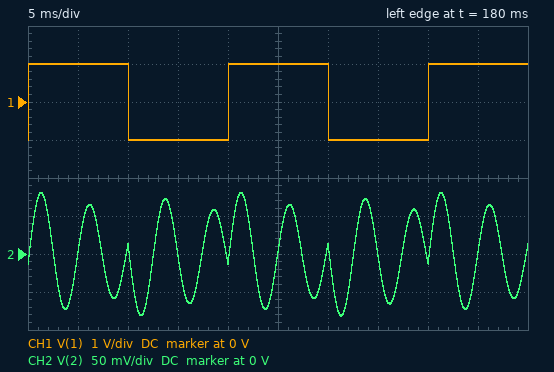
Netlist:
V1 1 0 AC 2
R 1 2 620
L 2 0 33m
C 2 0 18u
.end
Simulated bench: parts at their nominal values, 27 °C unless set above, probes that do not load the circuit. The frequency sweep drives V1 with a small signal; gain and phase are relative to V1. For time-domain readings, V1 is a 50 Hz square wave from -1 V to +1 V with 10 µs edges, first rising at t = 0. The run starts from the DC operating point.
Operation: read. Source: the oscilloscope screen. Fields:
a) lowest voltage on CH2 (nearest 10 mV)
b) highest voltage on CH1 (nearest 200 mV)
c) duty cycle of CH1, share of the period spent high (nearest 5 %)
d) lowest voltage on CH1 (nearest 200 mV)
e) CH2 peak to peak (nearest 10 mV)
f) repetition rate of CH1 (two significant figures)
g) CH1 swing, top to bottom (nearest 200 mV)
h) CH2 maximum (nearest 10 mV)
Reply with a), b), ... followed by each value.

a) -80 mV
b) 1.0 V
c) 50 %
d) -1.0 V
e) 160 mV
f) 50 Hz
g) 2.0 V
h) 80 mV
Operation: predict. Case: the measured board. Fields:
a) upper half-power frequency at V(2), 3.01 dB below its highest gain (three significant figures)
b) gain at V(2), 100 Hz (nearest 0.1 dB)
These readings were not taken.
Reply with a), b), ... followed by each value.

a) 214 Hz
b) -27.2 dB
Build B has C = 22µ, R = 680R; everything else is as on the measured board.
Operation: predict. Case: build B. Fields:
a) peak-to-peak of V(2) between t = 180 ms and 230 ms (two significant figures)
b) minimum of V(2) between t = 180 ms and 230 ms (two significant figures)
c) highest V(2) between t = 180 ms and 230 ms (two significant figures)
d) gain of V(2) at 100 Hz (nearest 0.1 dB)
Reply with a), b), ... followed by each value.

a) 140 mV
b) -70 mV
c) 70 mV
d) -27.4 dB
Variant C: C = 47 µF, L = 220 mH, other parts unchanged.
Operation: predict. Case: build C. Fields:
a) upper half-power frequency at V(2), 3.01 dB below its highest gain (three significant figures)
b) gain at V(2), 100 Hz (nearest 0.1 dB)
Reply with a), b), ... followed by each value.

a) 52.3 Hz
b) -22.8 dB
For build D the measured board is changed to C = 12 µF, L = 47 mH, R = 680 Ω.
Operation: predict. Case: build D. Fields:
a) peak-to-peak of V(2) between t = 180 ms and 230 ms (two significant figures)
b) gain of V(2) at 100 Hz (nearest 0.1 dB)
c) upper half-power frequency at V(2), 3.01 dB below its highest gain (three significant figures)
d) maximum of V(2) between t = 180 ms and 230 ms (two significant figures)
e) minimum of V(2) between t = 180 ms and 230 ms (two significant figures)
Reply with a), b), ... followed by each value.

a) 230 mV
b) -25.1 dB
c) 222 Hz
d) 120 mV
e) -120 mV
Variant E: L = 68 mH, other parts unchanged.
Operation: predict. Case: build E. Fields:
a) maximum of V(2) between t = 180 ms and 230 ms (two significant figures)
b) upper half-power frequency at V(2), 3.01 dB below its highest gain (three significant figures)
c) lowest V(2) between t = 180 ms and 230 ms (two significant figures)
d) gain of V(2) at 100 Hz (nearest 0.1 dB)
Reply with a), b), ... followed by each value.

a) 370 mV
b) 151 Hz
c) -370 mV
d) -17.6 dB
